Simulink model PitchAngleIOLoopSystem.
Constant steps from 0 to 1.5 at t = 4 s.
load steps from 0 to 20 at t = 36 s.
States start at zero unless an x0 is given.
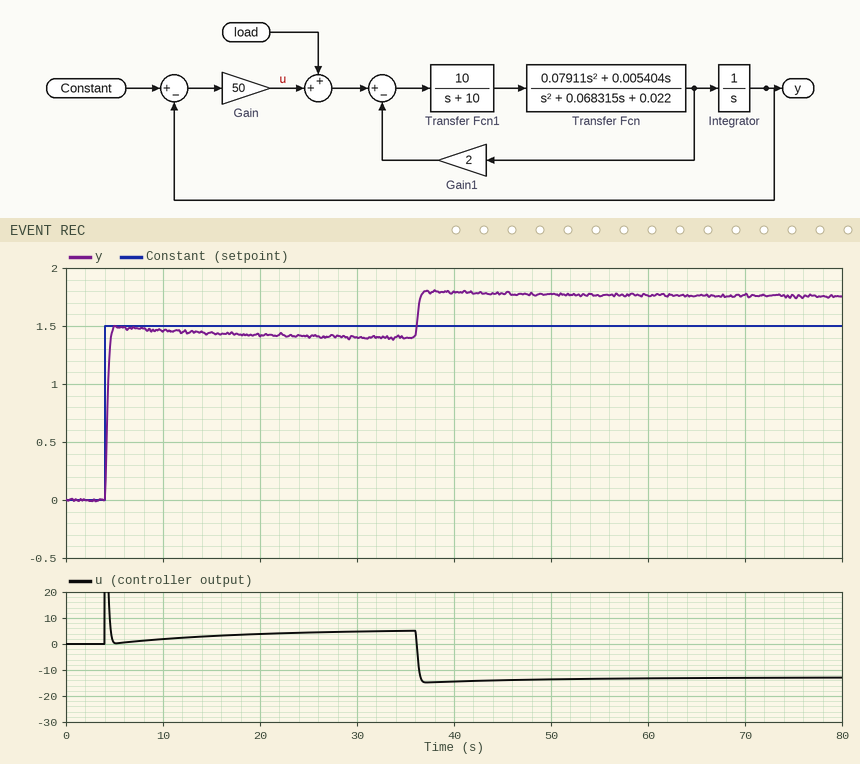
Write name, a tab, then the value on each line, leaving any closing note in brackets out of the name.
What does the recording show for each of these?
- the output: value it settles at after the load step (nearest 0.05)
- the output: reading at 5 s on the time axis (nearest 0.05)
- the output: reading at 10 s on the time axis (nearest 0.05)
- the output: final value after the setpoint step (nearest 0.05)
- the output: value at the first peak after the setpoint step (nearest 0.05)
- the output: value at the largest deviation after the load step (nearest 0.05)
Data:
the output: value it settles at after the load step	1.75
the output: reading at 5 s on the time axis	1.50
the output: reading at 10 s on the time axis	1.45
the output: final value after the setpoint step	1.40
the output: value at the first peak after the setpoint step	1.50
the output: value at the largest deviation after the load step	1.80
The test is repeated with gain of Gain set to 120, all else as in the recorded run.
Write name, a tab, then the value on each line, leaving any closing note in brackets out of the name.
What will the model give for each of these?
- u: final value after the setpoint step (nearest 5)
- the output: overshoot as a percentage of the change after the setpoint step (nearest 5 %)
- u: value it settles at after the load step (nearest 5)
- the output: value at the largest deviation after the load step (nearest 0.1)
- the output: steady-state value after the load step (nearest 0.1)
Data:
u: final value after the setpoint step	5
the output: overshoot as a percentage of the change after the setpoint step	15 %
u: value it settles at after the load step	-15
the output: value at the largest deviation after the load step	1.6
the output: steady-state value after the load step	1.6
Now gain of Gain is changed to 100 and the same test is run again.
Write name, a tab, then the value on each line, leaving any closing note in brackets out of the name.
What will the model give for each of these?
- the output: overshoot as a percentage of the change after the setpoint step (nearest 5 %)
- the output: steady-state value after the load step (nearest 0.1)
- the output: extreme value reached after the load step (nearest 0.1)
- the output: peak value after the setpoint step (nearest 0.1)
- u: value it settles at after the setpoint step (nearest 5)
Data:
the output: overshoot as a percentage of the change after the setpoint step	10 %
the output: steady-state value after the load step	1.6
the output: extreme value reached after the load step	1.7
the output: peak value after the setpoint step	1.6
u: value it settles at after the setpoint step	5
